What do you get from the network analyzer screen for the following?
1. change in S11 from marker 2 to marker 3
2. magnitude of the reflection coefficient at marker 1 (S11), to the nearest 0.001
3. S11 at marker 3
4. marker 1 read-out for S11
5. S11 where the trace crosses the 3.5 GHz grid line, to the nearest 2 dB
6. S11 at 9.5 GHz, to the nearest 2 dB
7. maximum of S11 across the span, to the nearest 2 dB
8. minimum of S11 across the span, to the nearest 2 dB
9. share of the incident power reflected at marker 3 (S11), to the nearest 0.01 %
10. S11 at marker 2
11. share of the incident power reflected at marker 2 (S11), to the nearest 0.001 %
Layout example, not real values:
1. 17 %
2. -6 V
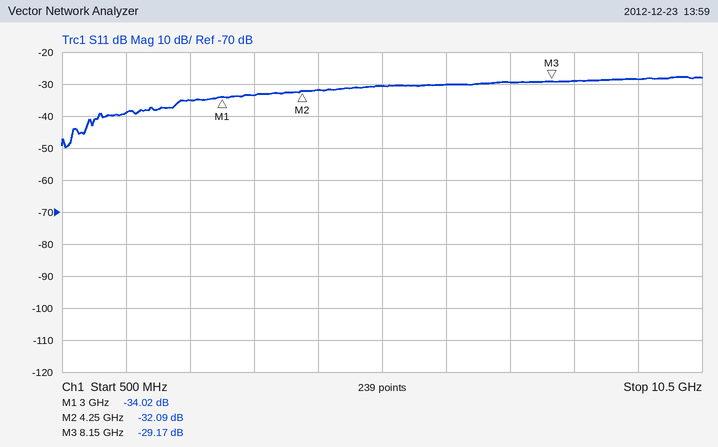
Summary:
1. 2.92 dB
2. 0.020
3. -29.17 dB
4. -34.02 dB
5. -34 dB
6. -28 dB
7. -28 dB
8. -50 dB
9. 0.12 %
10. -32.09 dB
11. 0.062 %
